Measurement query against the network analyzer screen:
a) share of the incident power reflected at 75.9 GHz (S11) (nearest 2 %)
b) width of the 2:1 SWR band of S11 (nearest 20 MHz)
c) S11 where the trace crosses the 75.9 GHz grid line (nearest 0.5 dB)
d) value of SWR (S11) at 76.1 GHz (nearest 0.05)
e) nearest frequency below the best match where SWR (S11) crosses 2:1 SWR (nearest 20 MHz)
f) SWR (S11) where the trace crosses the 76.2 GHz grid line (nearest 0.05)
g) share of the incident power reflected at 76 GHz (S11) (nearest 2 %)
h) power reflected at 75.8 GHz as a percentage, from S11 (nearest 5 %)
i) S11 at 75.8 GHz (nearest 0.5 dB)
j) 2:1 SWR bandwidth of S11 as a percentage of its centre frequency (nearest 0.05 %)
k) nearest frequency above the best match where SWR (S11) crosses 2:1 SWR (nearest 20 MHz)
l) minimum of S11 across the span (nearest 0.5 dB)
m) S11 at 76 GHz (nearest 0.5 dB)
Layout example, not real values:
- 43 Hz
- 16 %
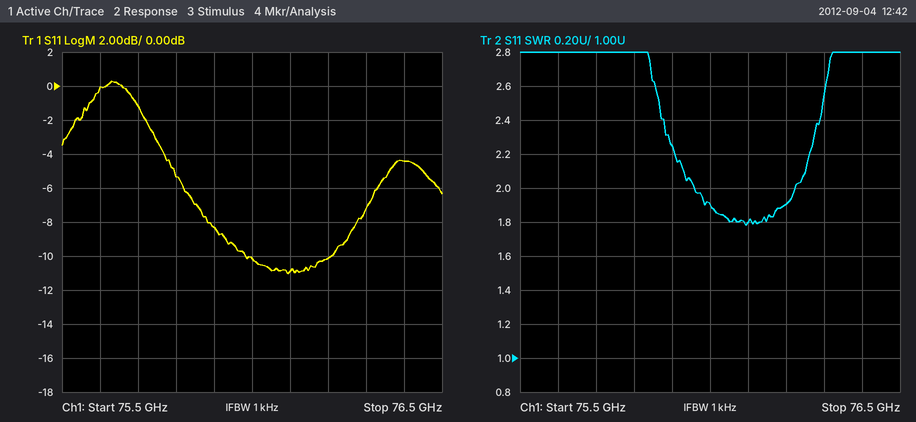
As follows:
- 14 %
- 260 MHz
- -8.5 dB
- 1.80
- 75.96 GHz
- 1.90
- 10 %
- 30 %
- -5.5 dB
- 0.35 %
- 76.22 GHz
- -11.0 dB
- -10.0 dB
